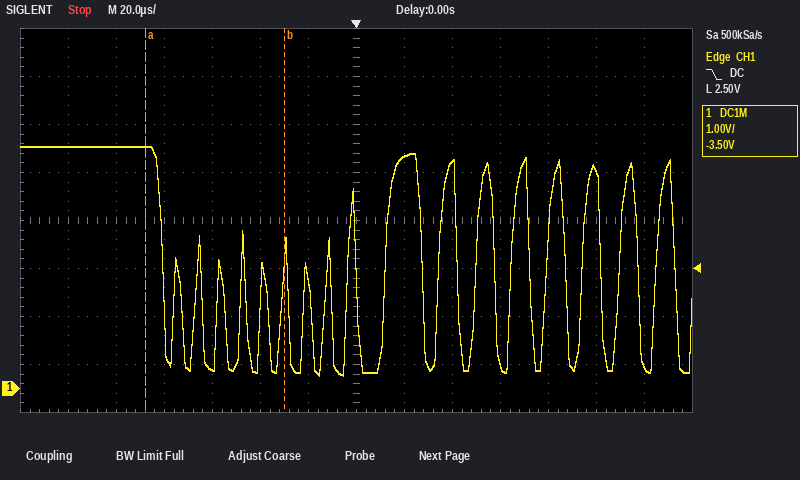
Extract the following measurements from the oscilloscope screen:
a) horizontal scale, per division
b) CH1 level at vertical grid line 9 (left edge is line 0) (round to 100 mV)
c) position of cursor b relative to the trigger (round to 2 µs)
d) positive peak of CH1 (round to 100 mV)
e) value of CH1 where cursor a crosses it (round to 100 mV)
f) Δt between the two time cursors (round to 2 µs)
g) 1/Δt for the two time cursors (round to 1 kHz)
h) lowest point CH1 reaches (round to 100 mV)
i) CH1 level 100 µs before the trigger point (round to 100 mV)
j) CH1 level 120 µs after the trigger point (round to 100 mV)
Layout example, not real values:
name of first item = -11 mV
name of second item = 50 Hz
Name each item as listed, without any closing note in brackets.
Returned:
horizontal scale, per division = 20 µs
CH1 level at vertical grid line 9 (left edge is line 0) = 4.7 V
position of cursor b relative to the trigger = -30 µs
positive peak of CH1 = 5.0 V
value of CH1 where cursor a crosses it = 5.0 V
Δt between the two time cursors = 58 µs
1/Δt for the two time cursors = 17 kHz
lowest point CH1 reaches = 300 mV
CH1 level 100 µs before the trigger point = 5.0 V
CH1 level 120 µs after the trigger point = 500 mV
